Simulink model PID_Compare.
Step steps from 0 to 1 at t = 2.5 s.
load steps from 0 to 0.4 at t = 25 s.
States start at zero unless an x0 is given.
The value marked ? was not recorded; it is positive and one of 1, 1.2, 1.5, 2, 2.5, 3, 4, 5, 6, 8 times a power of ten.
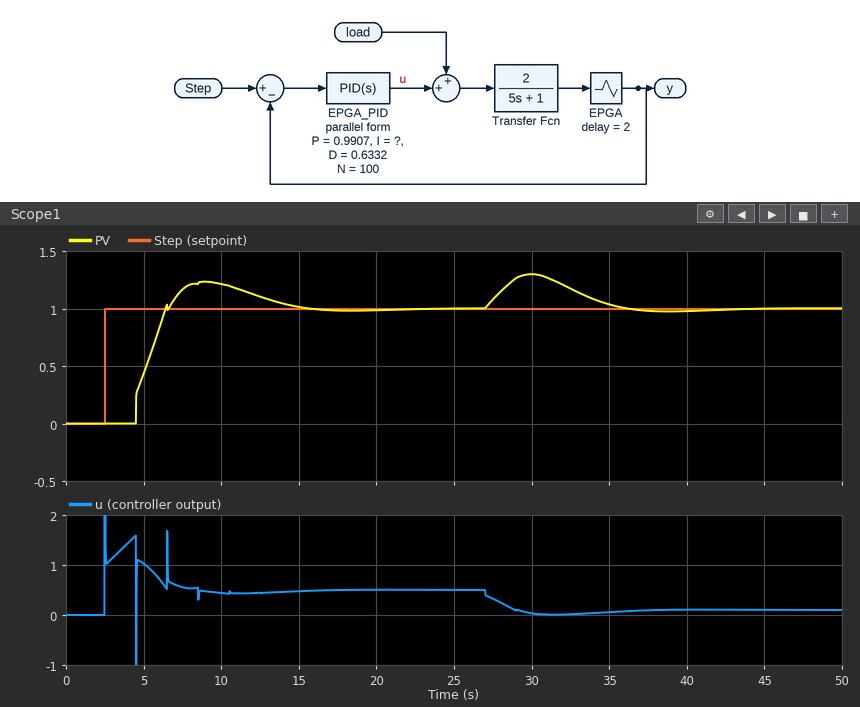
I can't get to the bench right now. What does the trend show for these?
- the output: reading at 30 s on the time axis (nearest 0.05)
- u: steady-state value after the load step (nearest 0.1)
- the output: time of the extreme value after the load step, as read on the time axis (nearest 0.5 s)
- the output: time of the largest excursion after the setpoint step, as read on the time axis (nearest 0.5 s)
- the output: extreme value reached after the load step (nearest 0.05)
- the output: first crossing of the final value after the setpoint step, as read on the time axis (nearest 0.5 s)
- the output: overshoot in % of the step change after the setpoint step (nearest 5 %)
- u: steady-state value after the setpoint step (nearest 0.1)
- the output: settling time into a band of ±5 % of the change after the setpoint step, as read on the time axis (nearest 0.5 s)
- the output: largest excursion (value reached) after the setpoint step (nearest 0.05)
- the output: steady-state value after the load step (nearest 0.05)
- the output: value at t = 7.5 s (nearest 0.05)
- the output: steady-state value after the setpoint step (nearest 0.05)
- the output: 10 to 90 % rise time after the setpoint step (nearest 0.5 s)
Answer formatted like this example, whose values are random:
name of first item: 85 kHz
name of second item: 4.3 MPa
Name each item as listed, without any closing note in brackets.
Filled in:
the output: reading at 30 s on the time axis: 1.30
u: steady-state value after the load step: 0.1
the output: time of the extreme value after the load step, as read on the time axis: 30.0 s
the output: time of the largest excursion after the setpoint step, as read on the time axis: 9.0 s
the output: extreme value reached after the load step: 1.30
the output: first crossing of the final value after the setpoint step, as read on the time axis: 6.5 s
the output: overshoot in % of the step change after the setpoint step: 25 %
u: steady-state value after the setpoint step: 0.5
the output: settling time into a band of ±5 % of the change after the setpoint step, as read on the time axis: 14.0 s
the output: largest excursion (value reached) after the setpoint step: 1.25
the output: steady-state value after the load step: 1.00
the output: value at t = 7.5 s: 1.15
the output: steady-state value after the setpoint step: 1.00
the output: 10 to 90 % rise time after the setpoint step: 1.5 s
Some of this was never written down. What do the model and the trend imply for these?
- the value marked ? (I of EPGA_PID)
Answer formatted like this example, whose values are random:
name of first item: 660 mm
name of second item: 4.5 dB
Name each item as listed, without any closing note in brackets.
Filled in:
the value marked ?: 0.3
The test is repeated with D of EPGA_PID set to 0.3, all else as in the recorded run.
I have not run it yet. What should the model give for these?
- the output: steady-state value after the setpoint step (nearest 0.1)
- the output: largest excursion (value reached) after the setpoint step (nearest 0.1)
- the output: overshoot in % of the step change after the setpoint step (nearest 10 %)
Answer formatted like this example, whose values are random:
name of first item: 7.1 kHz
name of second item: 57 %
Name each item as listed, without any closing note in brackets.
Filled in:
the output: steady-state value after the setpoint step: 1.0
the output: largest excursion (value reached) after the setpoint step: 1.4
the output: overshoot in % of the step change after the setpoint step: 40 %
